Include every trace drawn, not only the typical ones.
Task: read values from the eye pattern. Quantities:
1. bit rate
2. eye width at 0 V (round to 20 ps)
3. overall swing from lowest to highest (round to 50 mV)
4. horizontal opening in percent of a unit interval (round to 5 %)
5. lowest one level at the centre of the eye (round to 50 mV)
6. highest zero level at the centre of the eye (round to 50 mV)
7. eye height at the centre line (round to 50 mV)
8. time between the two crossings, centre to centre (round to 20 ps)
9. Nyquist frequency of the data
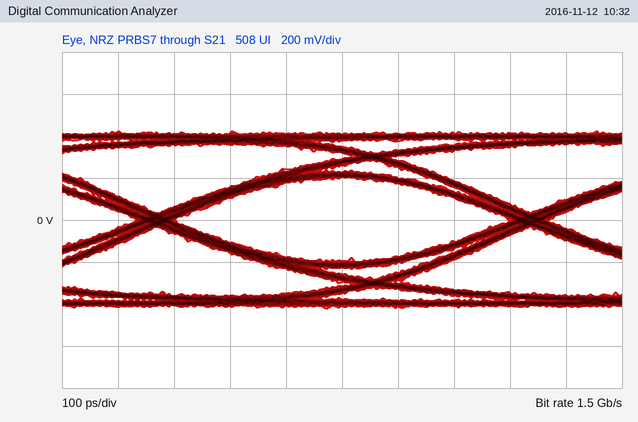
1.5 Gb/s
600 ps
850 mV
90 %
200 mV
-200 mV
400 mV
660 ps
750 MHz
